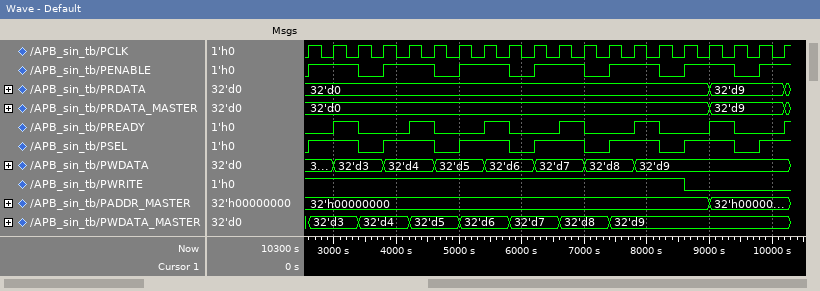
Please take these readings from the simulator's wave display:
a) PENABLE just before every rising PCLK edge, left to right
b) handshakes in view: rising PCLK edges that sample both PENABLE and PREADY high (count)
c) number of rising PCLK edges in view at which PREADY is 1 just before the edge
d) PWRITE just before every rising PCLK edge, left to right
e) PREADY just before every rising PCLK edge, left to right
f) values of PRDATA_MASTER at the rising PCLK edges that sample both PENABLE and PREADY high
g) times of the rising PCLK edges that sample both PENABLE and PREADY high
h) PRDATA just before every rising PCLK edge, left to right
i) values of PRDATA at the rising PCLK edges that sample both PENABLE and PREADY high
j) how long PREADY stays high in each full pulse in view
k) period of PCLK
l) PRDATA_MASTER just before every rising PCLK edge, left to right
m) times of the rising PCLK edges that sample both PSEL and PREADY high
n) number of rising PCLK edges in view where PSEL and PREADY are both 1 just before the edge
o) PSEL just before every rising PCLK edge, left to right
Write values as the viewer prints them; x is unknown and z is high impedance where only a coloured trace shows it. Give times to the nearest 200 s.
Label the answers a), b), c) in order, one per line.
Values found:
a) 0 1 1 0 1 1 0 1 1 0 1 1 0 1 1 0 1 1 0 1
b) 6
c) 6
d) 1 1 1 1 1 1 1 1 1 1 1 1 1 1 1 1 0 0 0 0
e) 0 0 1 0 0 1 0 0 1 0 0 1 0 0 1 0 0 1 0 0
f) 32'd0, 32'd0, 32'd0, 32'd0, 32'd0, 32'd9
g) 3400 s, 4600 s, 5800 s, 7000 s, 8200 s, 9400 s
h) 32'd0, 32'd0, 32'd0, 32'd0, 32'd0, 32'd0, 32'd0, 32'd0, 32'd0, 32'd0, 32'd0, 32'd0, 32'd0, 32'd0, 32'd0, 32'd0, 32'd0, 32'd9, 32'd9, 32'd9
i) 32'd0, 32'd0, 32'd0, 32'd0, 32'd0, 32'd9
j) 400 s, 400 s, 400 s, 400 s, 400 s, 400 s
k) 400 s
l) 32'd0, 32'd0, 32'd0, 32'd0, 32'd0, 32'd0, 32'd0, 32'd0, 32'd0, 32'd0, 32'd0, 32'd0, 32'd0, 32'd0, 32'd0, 32'd0, 32'd0, 32'd9, 32'd9, 32'd9
m) 3400 s, 4600 s, 5800 s, 7000 s, 8200 s, 9400 s
n) 6
o) 0 1 1 0 1 1 0 1 1 0 1 1 0 1 1 0 1 1 0 1
